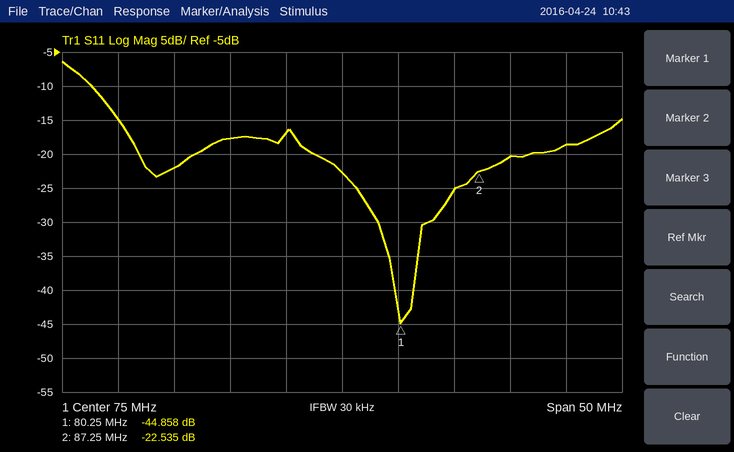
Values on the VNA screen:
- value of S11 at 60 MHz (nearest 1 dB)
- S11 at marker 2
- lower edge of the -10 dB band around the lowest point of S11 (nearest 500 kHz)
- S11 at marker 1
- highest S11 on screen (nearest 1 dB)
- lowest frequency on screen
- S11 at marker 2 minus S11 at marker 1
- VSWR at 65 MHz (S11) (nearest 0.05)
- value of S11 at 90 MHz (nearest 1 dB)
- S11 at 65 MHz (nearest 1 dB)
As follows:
-22 dB
-22.535 dB
52.5 MHz
-44.858 dB
-6 dB
50 MHz
22.323 dB
1.30
-20 dB
-18 dB
